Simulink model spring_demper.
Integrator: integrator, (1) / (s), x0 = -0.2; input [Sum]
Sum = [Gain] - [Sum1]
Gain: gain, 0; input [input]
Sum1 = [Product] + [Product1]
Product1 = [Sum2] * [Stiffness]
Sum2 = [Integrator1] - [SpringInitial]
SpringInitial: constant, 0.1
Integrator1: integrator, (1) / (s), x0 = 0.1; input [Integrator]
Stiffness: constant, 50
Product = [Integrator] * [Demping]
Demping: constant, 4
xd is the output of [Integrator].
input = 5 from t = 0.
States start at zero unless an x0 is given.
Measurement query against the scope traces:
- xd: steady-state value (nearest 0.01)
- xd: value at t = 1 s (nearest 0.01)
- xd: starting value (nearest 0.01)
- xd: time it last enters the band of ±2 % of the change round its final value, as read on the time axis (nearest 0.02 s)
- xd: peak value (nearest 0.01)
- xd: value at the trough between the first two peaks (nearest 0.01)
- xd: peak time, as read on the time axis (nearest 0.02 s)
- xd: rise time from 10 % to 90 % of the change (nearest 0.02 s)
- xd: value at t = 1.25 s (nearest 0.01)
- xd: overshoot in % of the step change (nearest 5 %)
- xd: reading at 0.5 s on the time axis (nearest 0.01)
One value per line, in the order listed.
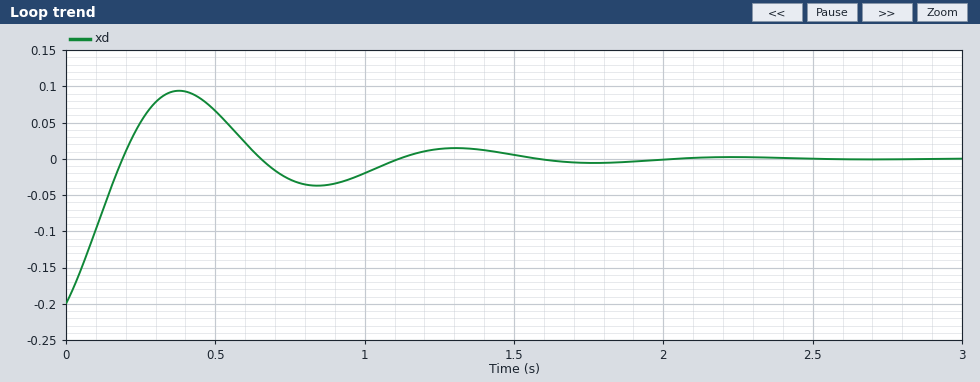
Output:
0.00
-0.02
-0.20
1.90 s
0.09
-0.04
0.38 s
0.14 s
0.01
45 %
0.07
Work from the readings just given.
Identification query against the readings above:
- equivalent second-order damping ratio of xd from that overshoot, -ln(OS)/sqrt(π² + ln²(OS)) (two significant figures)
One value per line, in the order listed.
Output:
0.25
